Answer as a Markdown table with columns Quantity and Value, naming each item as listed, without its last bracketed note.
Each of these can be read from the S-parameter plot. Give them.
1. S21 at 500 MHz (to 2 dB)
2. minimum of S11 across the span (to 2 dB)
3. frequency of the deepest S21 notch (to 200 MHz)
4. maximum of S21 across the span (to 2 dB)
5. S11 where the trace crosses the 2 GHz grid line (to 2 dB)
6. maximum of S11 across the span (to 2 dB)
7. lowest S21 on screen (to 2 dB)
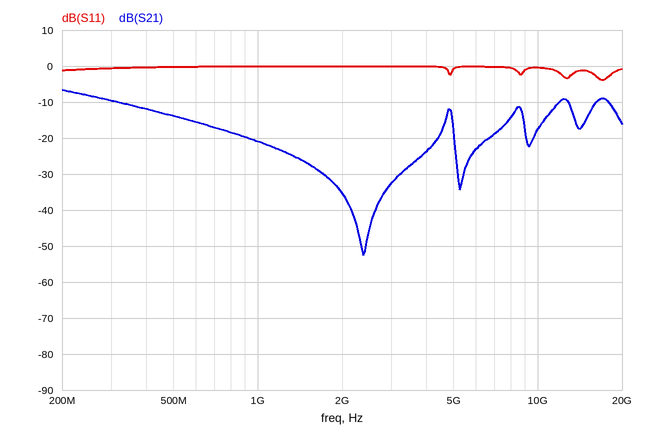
| Quantity | Value |
|---|---|
| S21 at 500 MHz | -14 dB |
| minimum of S11 across the span | -4 dB |
| frequency of the deepest S21 notch | 2.4 GHz |
| maximum of S21 across the span | -6 dB |
| S11 where the trace crosses the 2 GHz grid line | 0 dB |
| maximum of S11 across the span | 0 dB |
| lowest S21 on screen | -52 dB |
